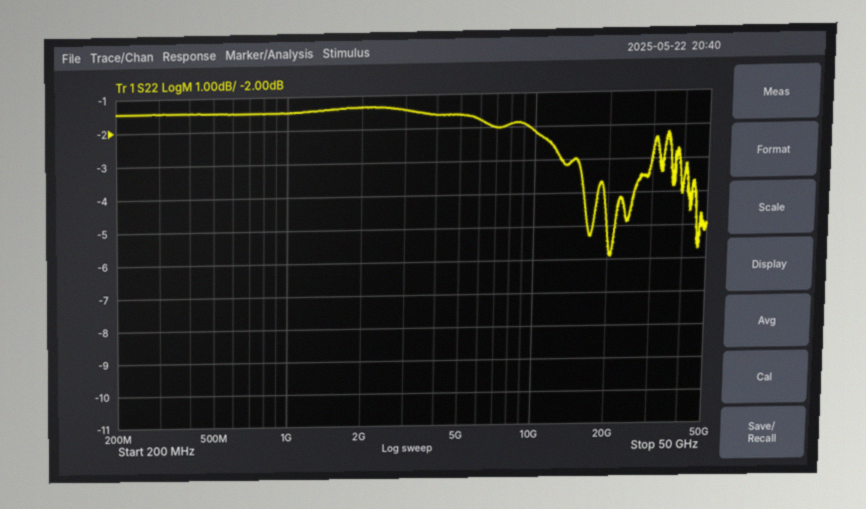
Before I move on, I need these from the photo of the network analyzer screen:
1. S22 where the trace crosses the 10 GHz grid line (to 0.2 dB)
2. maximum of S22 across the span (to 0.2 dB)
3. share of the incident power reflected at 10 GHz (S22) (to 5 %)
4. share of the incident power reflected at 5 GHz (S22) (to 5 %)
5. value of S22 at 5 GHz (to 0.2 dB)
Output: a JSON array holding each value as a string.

["-2.2 dB", "-1.4 dB", "60 %", "70 %", "-1.6 dB"]
